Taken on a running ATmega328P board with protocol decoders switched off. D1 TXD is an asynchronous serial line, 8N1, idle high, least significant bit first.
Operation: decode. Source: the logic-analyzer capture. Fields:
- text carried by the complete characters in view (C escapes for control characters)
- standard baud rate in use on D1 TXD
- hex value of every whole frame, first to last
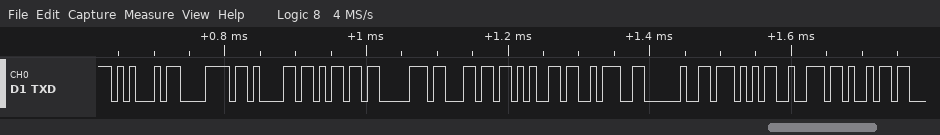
"Example: Wri"
115200 baud
0x45 0x78 0x61 0x6D 0x70 0x6C 0x65 0x3A 0x20 0x57 0x72 0x69
